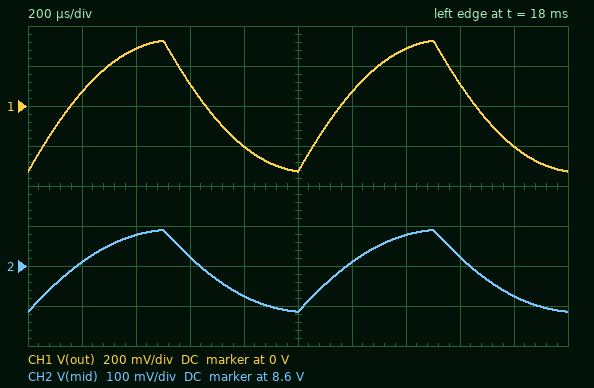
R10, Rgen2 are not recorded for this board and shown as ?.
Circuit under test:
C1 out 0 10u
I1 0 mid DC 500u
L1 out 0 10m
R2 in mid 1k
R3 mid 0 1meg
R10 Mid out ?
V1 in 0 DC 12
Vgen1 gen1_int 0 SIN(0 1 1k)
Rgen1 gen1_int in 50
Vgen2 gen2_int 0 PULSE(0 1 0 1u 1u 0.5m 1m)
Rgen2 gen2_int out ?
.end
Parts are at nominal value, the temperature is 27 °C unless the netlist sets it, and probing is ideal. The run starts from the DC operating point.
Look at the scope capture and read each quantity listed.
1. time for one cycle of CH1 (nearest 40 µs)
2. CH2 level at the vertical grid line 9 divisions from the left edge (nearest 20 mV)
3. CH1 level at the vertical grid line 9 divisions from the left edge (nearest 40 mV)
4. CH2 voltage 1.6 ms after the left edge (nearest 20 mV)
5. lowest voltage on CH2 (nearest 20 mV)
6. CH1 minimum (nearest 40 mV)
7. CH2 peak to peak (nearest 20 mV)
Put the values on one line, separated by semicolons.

1.00 ms; 8.52 V; -200 mV; 8.62 V; 8.48 V; -320 mV; 200 mV
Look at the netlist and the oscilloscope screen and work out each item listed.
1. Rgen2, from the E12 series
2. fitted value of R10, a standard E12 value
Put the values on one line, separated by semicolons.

39 Ω; 2.2 kΩ
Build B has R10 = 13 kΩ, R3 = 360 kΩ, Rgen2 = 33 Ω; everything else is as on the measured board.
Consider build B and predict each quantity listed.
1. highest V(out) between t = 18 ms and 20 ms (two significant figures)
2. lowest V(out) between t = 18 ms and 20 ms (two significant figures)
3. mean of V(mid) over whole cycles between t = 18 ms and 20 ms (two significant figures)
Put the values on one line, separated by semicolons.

360 mV; -360 mV; 12 V
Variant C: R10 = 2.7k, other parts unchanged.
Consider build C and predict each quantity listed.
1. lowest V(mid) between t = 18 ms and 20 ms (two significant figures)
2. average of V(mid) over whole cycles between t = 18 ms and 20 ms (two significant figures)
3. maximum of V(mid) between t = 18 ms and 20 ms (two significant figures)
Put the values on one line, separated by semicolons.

9.0 V; 9.1 V; 9.2 V
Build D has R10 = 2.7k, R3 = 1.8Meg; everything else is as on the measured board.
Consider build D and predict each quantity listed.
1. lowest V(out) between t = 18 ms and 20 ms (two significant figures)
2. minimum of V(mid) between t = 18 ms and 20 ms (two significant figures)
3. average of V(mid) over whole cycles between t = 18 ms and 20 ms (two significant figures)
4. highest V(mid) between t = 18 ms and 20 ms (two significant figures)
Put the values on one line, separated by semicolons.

-330 mV; 9.0 V; 9.1 V; 9.2 V
